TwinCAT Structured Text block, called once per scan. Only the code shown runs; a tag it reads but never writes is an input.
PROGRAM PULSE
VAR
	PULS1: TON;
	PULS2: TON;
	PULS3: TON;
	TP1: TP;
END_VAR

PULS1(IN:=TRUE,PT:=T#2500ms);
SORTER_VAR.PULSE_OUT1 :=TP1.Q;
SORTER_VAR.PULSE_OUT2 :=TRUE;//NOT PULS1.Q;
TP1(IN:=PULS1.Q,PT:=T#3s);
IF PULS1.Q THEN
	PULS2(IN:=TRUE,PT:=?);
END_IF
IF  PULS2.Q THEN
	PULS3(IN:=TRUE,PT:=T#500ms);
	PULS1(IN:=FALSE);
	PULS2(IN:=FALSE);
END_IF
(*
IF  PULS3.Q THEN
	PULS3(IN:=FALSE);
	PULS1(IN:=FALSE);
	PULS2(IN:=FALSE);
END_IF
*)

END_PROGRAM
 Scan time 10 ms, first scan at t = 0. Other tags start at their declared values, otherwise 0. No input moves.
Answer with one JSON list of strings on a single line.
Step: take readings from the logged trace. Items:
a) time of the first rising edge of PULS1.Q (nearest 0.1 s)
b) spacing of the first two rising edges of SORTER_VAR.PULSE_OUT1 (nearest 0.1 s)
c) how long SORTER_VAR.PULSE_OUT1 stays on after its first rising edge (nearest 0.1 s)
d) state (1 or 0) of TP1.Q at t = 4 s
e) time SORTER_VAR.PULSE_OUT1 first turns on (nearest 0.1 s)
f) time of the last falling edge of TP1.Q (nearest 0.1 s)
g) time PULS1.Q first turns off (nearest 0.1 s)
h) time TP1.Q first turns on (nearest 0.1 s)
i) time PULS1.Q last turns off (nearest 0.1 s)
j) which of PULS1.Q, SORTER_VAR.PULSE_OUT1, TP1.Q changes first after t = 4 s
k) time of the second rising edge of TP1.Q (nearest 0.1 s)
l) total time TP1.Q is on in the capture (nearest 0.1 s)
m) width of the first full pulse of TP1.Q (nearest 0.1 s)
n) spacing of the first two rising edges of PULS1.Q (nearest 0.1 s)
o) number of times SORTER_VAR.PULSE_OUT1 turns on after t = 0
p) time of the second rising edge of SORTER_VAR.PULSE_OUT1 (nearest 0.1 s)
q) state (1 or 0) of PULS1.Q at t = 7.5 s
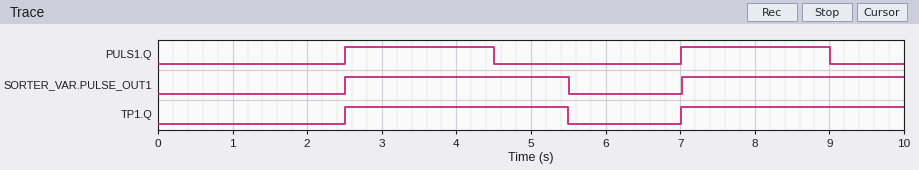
["2.5 s", "4.5 s", "3.0 s", "1", "2.5 s", "5.5 s", "4.5 s", "2.5 s", "9.0 s", "PULS1.Q", "7.0 s", "6.0 s", "3.0 s", "4.5 s", "2", "7.0 s", "1"]
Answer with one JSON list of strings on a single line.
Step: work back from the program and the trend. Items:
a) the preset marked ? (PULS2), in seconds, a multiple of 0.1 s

["2.0 s"]
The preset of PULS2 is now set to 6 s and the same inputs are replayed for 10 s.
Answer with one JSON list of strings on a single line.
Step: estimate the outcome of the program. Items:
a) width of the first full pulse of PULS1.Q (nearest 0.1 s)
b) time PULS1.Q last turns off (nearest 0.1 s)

["6.0 s", "8.5 s"]
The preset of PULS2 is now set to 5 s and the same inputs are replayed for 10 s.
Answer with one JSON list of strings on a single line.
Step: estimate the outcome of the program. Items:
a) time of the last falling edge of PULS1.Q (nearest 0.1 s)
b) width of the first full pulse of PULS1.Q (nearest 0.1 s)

["7.5 s", "5.0 s"]
